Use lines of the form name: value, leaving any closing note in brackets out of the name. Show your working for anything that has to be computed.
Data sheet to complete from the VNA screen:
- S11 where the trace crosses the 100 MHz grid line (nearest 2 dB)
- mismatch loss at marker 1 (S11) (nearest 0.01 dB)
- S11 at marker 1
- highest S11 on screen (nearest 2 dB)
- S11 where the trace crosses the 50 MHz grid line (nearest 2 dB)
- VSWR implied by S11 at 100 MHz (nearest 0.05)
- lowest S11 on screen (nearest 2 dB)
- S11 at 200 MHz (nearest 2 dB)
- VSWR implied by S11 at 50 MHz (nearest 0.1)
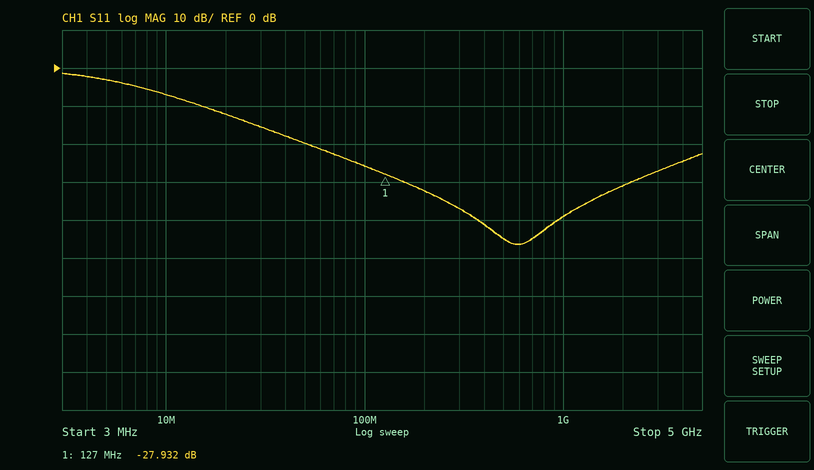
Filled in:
S11 where the trace crosses the 100 MHz grid line: -26 dB
mismatch loss at marker 1 (S11): −10 log10(1 − 10^(-27.932/10)) ≈ 0.01 dB
S11 at marker 1: -27.932 dB
highest S11 on screen: -2 dB
S11 where the trace crosses the 50 MHz grid line: -20 dB
VSWR implied by S11 at 100 MHz: |Γ| = 10^(-26/20) = 0.0501; VSWR = (1 + 0.0501)/(1 − 0.0501) ≈ 1.11, so 1.10 to the nearest 0.05
lowest S11 on screen: -46 dB
S11 at 200 MHz: -32 dB
VSWR implied by S11 at 50 MHz: |Γ| = 10^(-20/20) = 0.1000; VSWR = (1 + 0.1000)/(1 − 0.1000) ≈ 1.2
